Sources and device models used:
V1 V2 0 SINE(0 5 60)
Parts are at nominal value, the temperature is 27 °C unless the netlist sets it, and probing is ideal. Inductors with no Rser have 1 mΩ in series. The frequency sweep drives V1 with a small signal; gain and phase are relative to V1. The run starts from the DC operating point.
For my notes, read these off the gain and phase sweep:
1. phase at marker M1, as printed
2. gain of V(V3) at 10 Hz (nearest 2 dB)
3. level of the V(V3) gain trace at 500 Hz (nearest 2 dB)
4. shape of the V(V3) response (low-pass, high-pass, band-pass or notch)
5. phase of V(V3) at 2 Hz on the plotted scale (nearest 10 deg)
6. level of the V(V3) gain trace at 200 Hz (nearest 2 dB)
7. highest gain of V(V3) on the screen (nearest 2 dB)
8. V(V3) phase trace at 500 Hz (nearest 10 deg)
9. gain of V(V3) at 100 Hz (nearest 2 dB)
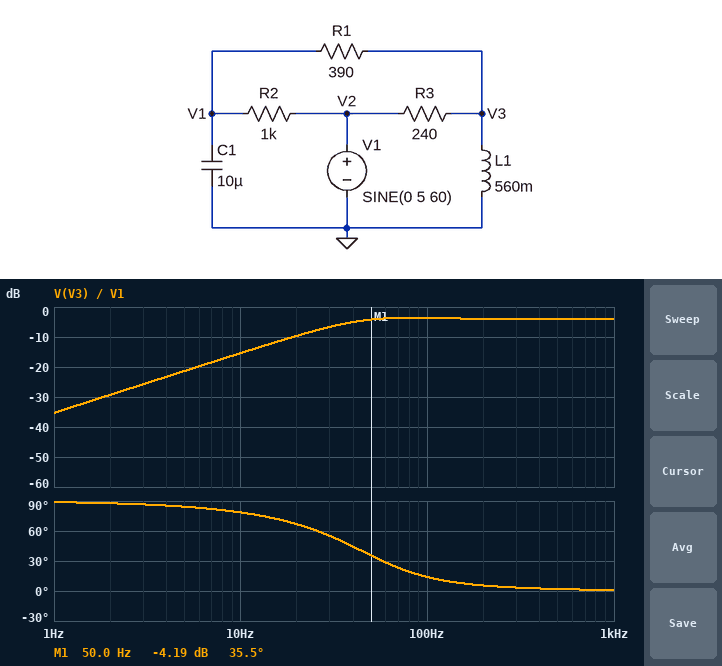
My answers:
35.5 deg
-16 dB
-4 dB
high-pass
90 deg
-4 dB
-4 dB
0 deg
-4 dB
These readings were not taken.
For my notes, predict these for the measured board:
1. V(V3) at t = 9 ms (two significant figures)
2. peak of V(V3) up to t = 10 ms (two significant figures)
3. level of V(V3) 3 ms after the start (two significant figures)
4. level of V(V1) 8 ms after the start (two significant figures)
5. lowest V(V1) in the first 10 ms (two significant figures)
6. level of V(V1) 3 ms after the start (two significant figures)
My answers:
-2.4 V
2.2 V
2.2 V
1.1 V
-550 mV
1.3 V
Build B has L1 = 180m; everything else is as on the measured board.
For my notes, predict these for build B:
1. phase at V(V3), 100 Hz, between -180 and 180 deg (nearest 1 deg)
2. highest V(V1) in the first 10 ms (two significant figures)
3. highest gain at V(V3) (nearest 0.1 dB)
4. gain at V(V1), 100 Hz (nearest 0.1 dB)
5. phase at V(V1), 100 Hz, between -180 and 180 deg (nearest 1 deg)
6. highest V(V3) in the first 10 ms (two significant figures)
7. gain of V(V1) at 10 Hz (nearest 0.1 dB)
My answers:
48 deg
1.4 V
-4.2 dB
-11.5 dB
-35 deg
1.1 V
-11.0 dB
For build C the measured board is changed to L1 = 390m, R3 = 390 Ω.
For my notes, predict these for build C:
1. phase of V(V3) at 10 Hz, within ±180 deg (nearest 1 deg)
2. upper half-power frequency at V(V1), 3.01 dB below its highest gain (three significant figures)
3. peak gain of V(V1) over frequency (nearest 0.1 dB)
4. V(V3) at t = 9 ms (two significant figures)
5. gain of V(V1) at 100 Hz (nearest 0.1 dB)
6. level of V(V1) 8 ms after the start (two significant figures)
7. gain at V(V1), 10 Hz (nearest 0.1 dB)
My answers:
83 deg
127 Hz
-8.8 dB
-1.8 V
-10.5 dB
800 mV
-10.8 dB
